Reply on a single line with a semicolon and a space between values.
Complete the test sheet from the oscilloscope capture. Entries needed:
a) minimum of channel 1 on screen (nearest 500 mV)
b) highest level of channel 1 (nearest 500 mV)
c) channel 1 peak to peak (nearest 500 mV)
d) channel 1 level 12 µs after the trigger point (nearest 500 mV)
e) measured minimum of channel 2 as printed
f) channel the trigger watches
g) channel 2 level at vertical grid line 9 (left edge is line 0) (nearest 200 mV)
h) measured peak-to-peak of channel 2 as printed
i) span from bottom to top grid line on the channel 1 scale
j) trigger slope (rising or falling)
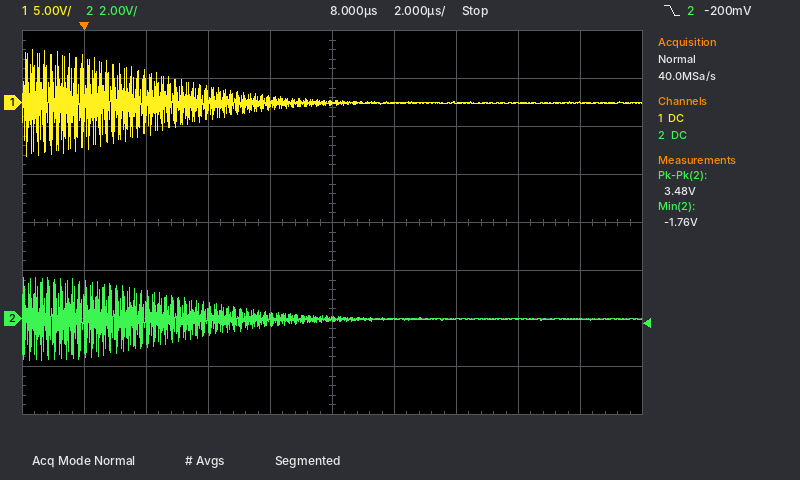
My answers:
-5.5 V; 5.5 V; 11.0 V; 0.0 V; -1.76 V; channel 2; 0.0 V; 3.48 V; 40 V; falling
